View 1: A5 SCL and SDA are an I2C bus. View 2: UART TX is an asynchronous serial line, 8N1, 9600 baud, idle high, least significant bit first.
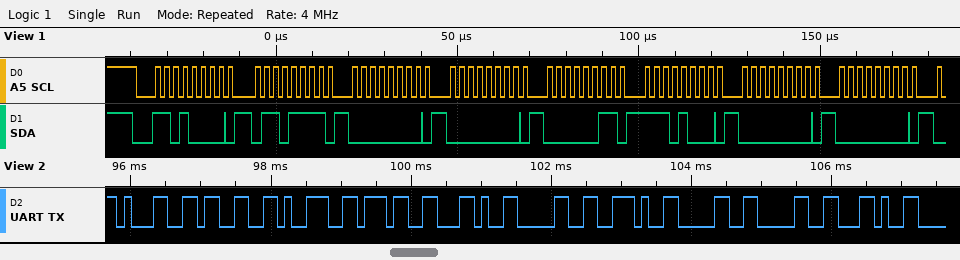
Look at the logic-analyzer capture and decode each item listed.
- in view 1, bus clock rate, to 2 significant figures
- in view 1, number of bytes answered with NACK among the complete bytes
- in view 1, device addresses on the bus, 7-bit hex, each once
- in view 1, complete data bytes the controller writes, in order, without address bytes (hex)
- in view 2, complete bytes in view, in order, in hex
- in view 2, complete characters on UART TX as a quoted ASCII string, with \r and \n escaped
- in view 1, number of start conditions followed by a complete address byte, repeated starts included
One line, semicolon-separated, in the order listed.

400 kHz; 0; 0x68; 6F 00 00 03 E8 00 00; 31 33 39 37 2C 30 2E 30 30 2C; "1397,0.00,"; 1
